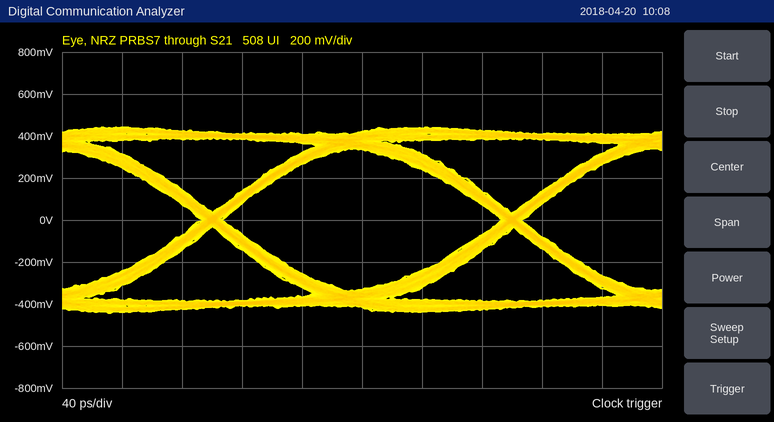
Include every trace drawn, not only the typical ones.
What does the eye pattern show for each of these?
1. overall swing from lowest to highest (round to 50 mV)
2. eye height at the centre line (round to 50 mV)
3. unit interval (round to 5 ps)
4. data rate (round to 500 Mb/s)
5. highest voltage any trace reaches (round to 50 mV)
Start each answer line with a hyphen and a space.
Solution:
- 900 mV
- 650 mV
- 200 ps
- 5.0 Gb/s
- 450 mV
